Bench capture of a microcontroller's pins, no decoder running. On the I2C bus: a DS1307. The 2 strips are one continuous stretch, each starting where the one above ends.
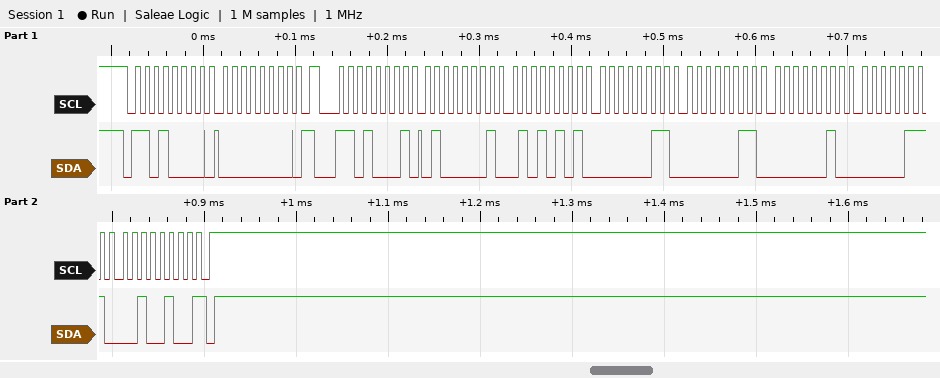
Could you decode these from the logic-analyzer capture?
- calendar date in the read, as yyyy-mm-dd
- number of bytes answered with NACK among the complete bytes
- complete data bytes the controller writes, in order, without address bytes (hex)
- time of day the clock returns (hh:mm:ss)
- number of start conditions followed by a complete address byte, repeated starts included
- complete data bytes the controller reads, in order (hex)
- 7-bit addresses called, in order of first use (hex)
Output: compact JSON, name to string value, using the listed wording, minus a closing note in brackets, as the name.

{"calendar date in the read, as yyyy-mm-dd": "2024-07-02", "number of bytes answered with NACK among the complete bytes": "1", "complete data bytes the controller writes, in order, without address bytes": "00", "time of day the clock returns": "03:55:41", "number of start conditions followed by a complete address byte, repeated starts included": "2", "complete data bytes the controller reads, in order": "41 55 03 03 02 07 24", "7-bit addresses called, in order of first use": "0x68"}
